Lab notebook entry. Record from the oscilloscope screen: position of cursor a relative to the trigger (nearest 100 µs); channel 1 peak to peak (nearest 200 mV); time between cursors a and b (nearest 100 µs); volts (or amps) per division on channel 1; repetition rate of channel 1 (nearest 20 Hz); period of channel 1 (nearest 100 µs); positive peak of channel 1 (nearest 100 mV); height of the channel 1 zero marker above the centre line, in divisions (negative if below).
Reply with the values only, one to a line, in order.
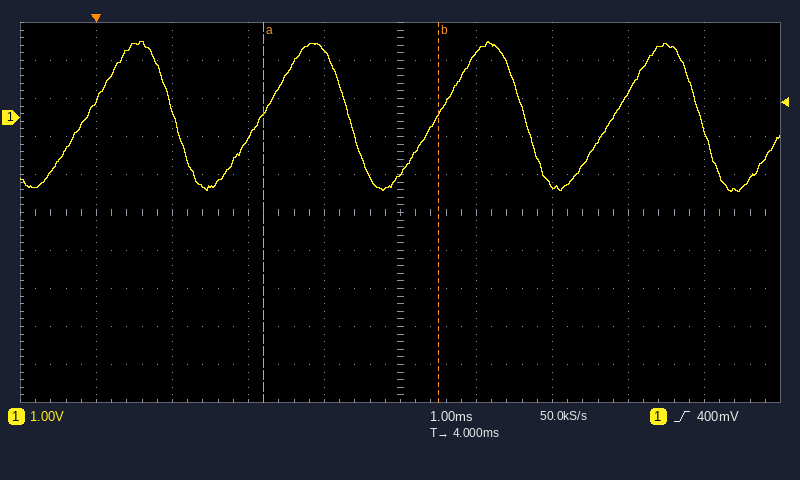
+2.2 ms
4.0 V
2.3 ms
1 V
440 Hz
2.3 ms
2.0 V
+2.5 div
